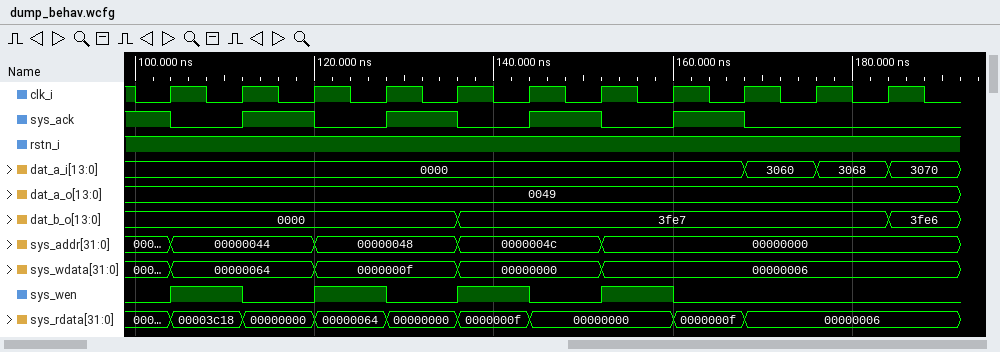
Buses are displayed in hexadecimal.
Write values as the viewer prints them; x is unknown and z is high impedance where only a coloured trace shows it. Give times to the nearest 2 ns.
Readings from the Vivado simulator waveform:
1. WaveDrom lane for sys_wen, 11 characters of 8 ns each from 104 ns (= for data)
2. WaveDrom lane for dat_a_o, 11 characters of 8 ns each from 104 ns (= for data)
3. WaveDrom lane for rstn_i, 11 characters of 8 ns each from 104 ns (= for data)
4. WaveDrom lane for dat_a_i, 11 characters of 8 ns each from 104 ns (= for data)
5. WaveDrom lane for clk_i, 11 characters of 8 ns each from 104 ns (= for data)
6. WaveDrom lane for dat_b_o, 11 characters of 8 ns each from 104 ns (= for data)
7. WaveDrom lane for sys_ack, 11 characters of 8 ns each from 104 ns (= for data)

{name: 'sys_wen', wave: '10101010...'}
{name: 'dat_a_o', wave: '=..........', data: '0049'}
{name: 'rstn_i', wave: '1..........'}
{name: 'dat_a_i', wave: '=.......===', data: '0000 3060 3068 3070'}
{name: 'clk_i', wave: 'p..........'}
{name: 'dat_b_o', wave: '=...=.....=', data: '0000 3fe7 3fe6'}
{name: 'sys_ack', wave: '010101010..'}
